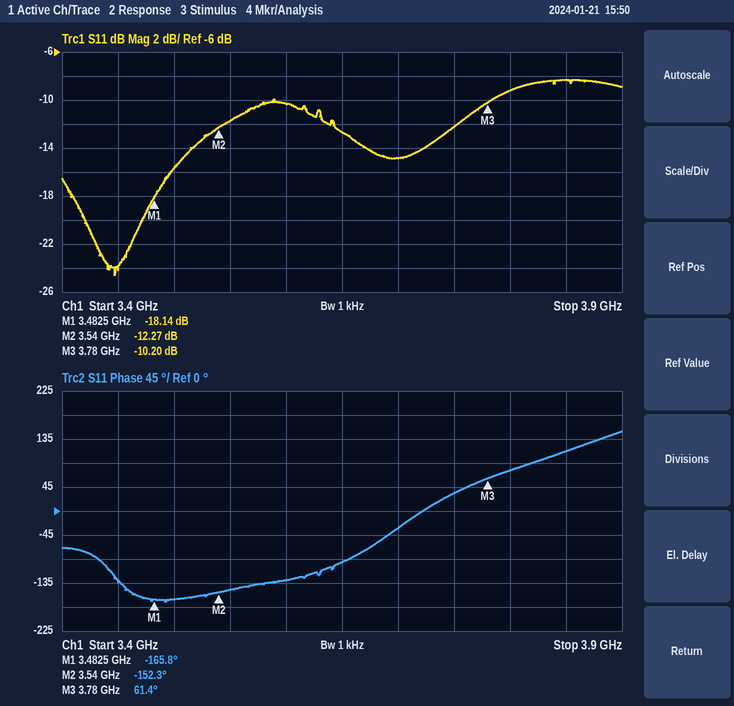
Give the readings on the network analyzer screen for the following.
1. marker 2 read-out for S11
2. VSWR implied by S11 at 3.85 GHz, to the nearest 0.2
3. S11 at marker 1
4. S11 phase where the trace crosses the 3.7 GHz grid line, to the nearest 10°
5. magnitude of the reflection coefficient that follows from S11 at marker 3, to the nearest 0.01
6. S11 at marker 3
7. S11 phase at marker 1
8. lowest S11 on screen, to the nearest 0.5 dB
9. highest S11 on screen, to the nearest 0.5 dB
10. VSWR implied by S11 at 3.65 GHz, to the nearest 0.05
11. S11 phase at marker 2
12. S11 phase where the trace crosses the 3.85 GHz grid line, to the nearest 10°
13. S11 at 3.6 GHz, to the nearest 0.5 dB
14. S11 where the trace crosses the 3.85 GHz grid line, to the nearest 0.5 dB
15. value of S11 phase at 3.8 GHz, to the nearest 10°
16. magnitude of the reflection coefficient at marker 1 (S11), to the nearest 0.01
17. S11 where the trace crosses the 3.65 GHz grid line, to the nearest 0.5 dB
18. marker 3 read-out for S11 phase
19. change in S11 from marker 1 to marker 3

-12.27 dB
2.2
-18.14 dB
-30°
0.31
-10.20 dB
-165.8°
-24.5 dB
-8.5 dB
1.60
-152.3°
110°
-10.5 dB
-8.5 dB
80°
0.12
-12.5 dB
61.4°
7.94 dB
